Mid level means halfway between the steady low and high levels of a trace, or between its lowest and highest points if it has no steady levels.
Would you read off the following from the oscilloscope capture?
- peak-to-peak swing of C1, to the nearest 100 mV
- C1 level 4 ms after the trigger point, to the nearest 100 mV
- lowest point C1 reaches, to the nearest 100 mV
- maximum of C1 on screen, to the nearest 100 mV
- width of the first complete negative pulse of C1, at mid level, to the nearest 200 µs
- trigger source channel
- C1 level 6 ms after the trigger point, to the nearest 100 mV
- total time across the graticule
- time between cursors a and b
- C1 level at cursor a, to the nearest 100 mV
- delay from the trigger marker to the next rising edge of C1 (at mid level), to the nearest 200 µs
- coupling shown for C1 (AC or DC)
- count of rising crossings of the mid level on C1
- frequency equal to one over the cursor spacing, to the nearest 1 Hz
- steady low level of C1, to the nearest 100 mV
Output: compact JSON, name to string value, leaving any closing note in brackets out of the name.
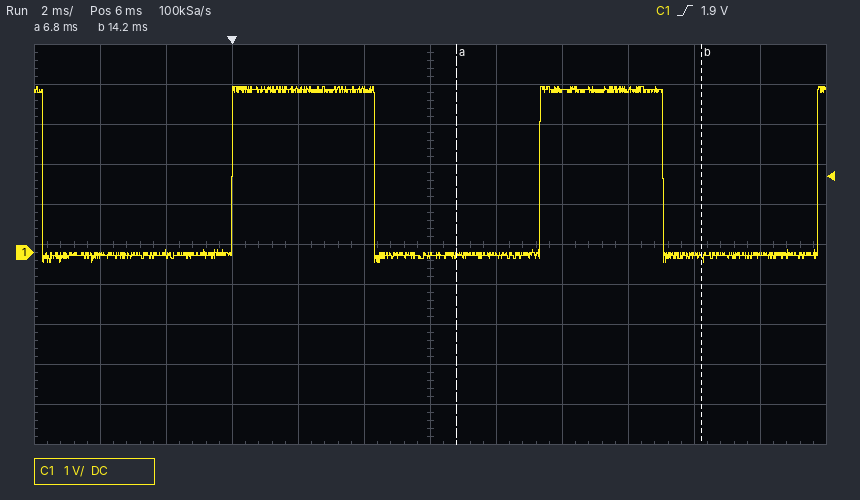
{"peak-to-peak swing of C1, to the nearest 100 mV": "4.4 V", "C1 level 4 ms after the trigger point, to the nearest 100 mV": "4.1 V", "lowest point C1 reaches, to the nearest 100 mV": "-200 mV", "maximum of C1 on screen, to the nearest 100 mV": "4.2 V", "width of the first complete negative pulse of C1, at mid level, to the nearest 200 µs": "5.8 ms", "trigger source channel": "C1", "C1 level 6 ms after the trigger point, to the nearest 100 mV": "-100 mV", "total time across the graticule": "24 ms", "time between cursors a and b": "7.4 ms", "C1 level at cursor a, to the nearest 100 mV": "-100 mV", "delay from the trigger marker to the next rising edge of C1 (at mid level), to the nearest 200 µs": "9.4 ms", "coupling shown for C1": "DC", "count of rising crossings of the mid level on C1": "3", "frequency equal to one over the cursor spacing, to the nearest 1 Hz": "135 Hz", "steady low level of C1, to the nearest 100 mV": "-100 mV"}
